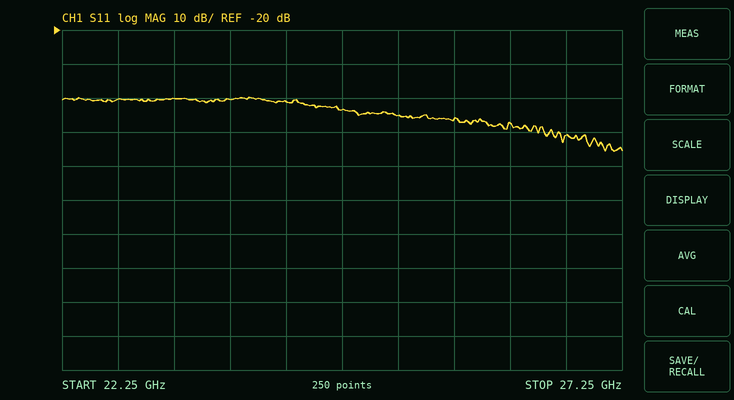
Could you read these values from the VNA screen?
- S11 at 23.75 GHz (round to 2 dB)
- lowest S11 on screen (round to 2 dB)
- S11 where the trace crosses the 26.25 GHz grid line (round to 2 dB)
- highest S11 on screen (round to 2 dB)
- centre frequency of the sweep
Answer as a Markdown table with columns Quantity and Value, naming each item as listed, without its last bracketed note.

| Quantity | Value |
|---|---|
| S11 at 23.75 GHz | -40 dB |
| lowest S11 on screen | -56 dB |
| S11 where the trace crosses the 26.25 GHz grid line | -48 dB |
| highest S11 on screen | -40 dB |
| centre frequency of the sweep | 24.75 GHz |
